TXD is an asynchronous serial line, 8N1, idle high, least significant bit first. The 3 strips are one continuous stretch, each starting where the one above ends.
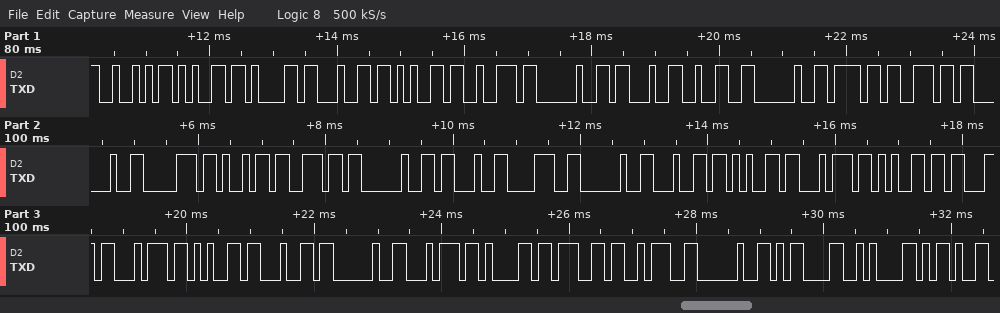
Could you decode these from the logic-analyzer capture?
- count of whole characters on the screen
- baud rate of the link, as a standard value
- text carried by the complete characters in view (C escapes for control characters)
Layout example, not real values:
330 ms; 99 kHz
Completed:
37; 9600 baud; "Reader #2 on pin #8 detected tag: \r\n-"
